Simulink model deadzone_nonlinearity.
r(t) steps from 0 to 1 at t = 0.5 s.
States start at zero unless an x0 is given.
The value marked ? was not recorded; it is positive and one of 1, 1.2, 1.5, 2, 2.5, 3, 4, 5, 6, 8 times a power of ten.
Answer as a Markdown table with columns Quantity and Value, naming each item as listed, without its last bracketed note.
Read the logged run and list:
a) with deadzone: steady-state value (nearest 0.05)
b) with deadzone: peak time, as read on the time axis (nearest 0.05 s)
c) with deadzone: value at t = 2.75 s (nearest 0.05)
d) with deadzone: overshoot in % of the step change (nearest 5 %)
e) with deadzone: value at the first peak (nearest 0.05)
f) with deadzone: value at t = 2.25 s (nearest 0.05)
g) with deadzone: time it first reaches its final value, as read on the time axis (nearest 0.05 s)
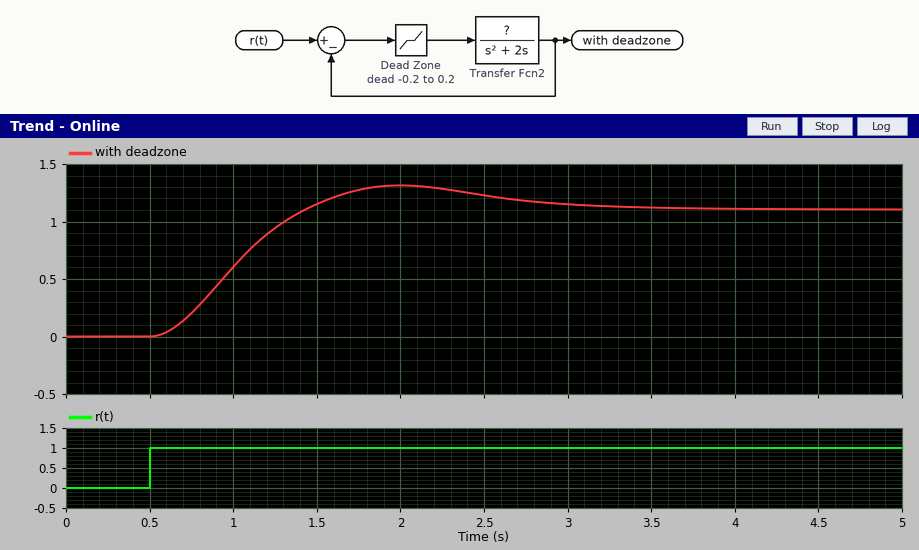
| Quantity | Value |
|---|---|
| with deadzone: steady-state value | 1.10 |
| with deadzone: peak time, as read on the time axis | 2.00 s |
| with deadzone: value at t = 2.75 s | 1.20 |
| with deadzone: overshoot in % of the step change | 20 % |
| with deadzone: value at the first peak | 1.30 |
| with deadzone: value at t = 2.25 s | 1.30 |
| with deadzone: time it first reaches its final value, as read on the time axis | 1.45 s |
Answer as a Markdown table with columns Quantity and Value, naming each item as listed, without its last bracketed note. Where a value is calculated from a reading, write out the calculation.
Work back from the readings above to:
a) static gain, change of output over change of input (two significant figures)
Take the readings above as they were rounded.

| Quantity | Value |
|---|---|
| static gain, change of output over change of input | (1.1 - 0) / (1 - 0) = 1.1 |
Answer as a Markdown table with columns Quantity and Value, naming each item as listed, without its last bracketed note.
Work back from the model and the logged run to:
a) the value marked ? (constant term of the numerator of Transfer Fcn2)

| Quantity | Value |
|---|---|
| the value marked ? | 10 |
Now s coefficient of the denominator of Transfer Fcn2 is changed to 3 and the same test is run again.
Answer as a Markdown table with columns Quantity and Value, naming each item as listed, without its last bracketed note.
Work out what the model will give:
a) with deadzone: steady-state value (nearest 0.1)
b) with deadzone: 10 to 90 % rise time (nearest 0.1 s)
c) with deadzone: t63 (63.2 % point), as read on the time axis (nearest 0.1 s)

| Quantity | Value |
|---|---|
| with deadzone: steady-state value | 1.1 |
| with deadzone: 10 to 90 % rise time | 0.9 s |
| with deadzone: t63 (63.2 % point), as read on the time axis | 1.1 s |
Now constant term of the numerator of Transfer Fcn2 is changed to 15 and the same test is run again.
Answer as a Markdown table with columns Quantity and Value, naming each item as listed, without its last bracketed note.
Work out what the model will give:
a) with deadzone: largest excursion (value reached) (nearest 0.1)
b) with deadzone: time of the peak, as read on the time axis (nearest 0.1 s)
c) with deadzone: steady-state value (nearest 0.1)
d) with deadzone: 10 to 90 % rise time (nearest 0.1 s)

| Quantity | Value |
|---|---|
| with deadzone: largest excursion (value reached) | 1.4 |
| with deadzone: time of the peak, as read on the time axis | 1.6 s |
| with deadzone: steady-state value | 1.0 |
| with deadzone: 10 to 90 % rise time | 0.4 s |
